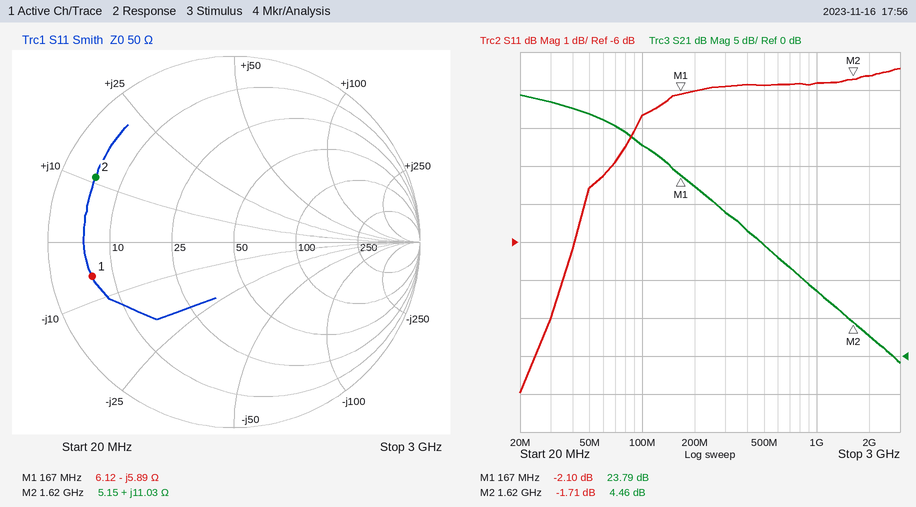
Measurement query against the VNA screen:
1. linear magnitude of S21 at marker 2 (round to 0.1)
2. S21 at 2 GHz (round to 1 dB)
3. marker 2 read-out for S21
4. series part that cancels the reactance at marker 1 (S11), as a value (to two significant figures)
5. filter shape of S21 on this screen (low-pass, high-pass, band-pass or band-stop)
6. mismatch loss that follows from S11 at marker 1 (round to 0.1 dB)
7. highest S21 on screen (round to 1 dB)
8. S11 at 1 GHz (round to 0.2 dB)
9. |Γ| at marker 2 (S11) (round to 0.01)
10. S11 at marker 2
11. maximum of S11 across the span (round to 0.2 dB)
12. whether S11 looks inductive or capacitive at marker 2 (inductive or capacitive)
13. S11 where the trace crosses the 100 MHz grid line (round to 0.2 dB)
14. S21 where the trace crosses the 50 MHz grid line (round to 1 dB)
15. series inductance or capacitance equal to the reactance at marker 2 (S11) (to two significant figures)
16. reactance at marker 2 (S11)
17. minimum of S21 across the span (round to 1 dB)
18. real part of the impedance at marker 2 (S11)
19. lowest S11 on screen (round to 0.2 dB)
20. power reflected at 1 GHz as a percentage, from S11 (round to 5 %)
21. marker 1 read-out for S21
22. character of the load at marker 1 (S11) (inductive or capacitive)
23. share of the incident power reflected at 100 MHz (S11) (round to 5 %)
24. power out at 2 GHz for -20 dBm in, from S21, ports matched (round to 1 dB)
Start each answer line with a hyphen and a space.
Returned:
- 1.7
- 3 dB
- 4.46 dB
- 5.6 nH
- low-pass
- 4.2 dB
- 34 dB
- -1.8 dB
- 0.82
- -1.71 dB
- -1.4 dB
- inductive
- -2.6 dB
- 32 dB
- 1.1 nH
- +11.03 Ω
- -1 dB
- 5.15 Ω
- -10.0 dB
- 65 %
- 23.79 dB
- capacitive
- 55 %
- -17 dBm
